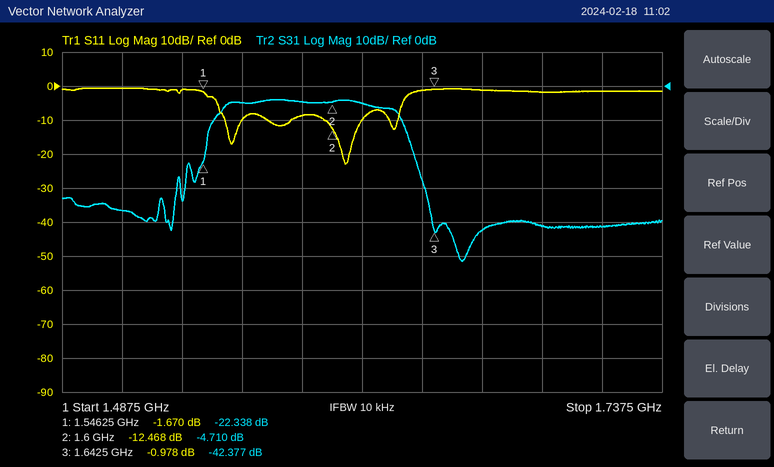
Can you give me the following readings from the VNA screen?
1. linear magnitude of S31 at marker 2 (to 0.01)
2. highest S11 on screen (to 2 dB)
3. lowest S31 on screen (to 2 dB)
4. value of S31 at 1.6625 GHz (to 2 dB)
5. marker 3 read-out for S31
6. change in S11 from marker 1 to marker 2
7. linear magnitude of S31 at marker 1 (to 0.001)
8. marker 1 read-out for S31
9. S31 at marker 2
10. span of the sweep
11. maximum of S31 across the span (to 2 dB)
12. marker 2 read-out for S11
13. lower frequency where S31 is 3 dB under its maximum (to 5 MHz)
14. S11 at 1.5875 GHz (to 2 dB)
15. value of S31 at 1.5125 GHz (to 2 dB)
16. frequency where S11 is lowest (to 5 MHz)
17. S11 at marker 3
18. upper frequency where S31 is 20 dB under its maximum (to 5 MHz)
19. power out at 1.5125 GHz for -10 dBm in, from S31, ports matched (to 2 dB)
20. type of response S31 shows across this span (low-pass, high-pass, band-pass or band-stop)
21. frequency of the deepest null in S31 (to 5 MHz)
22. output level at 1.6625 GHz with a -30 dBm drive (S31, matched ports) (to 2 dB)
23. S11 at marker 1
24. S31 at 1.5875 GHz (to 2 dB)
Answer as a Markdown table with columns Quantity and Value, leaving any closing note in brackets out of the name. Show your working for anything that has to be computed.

| Quantity | Value |
|---|---|
| linear magnitude of S31 at marker 2 | 10^(-4.71/20) ≈ 0.58 |
| highest S11 on screen | 0 dB |
| lowest S31 on screen | -52 dB |
| value of S31 at 1.6625 GHz | -42 dB |
| marker 3 read-out for S31 | -42.377 dB |
| change in S11 from marker 1 to marker 2 | -12.468 − (-1.67) = -10.798 dB |
| linear magnitude of S31 at marker 1 | 10^(-22.338/20) ≈ 0.076 |
| marker 1 read-out for S31 | -22.338 dB |
| S31 at marker 2 | -4.710 dB |
| span of the sweep | 250 MHz |
| maximum of S31 across the span | -4 dB |
| marker 2 read-out for S11 | -12.468 dB |
| lower frequency where S31 is 3 dB under its maximum | 1.555 GHz |
| S11 at 1.5875 GHz | -8 dB |
| value of S31 at 1.5125 GHz | -36 dB |
| frequency where S11 is lowest | 1.605 GHz |
| S11 at marker 3 | -0.978 dB |
| upper frequency where S31 is 20 dB under its maximum | 1.635 GHz |
| power out at 1.5125 GHz for -10 dBm in, from S31, ports matched | -10 dBm + (-36 dB) = -46 dBm |
| type of response S31 shows across this span | band-pass |
| frequency of the deepest null in S31 | 1.655 GHz |
| output level at 1.6625 GHz with a -30 dBm drive (S31, matched ports) | -30 dBm + (-42 dB) = -72 dBm |
| S11 at marker 1 | -1.670 dB |
| S31 at 1.5875 GHz | -4 dB |
